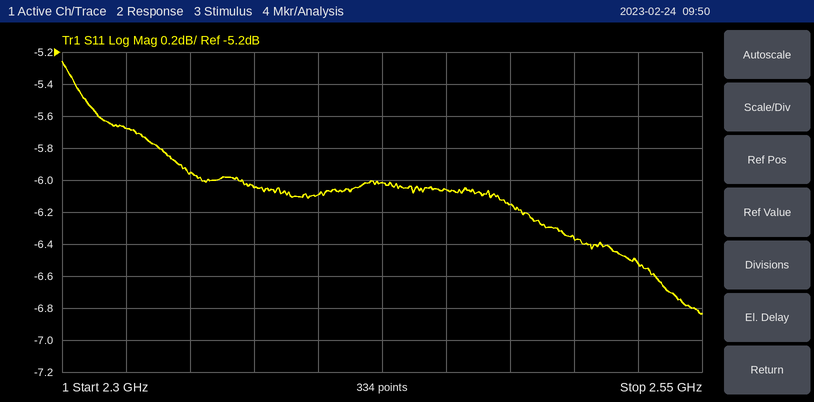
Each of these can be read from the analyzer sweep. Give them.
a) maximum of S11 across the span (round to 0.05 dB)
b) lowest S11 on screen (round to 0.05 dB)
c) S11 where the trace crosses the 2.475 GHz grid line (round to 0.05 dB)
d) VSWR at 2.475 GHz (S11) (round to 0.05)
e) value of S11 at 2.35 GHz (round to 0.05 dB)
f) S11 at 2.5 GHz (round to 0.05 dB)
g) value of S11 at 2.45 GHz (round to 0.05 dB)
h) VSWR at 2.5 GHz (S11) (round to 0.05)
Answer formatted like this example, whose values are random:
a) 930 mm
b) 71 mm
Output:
a) -5.25 dB
b) -6.85 dB
c) -6.15 dB
d) 2.95
e) -5.95 dB
f) -6.35 dB
g) -6.05 dB
h) 2.85
